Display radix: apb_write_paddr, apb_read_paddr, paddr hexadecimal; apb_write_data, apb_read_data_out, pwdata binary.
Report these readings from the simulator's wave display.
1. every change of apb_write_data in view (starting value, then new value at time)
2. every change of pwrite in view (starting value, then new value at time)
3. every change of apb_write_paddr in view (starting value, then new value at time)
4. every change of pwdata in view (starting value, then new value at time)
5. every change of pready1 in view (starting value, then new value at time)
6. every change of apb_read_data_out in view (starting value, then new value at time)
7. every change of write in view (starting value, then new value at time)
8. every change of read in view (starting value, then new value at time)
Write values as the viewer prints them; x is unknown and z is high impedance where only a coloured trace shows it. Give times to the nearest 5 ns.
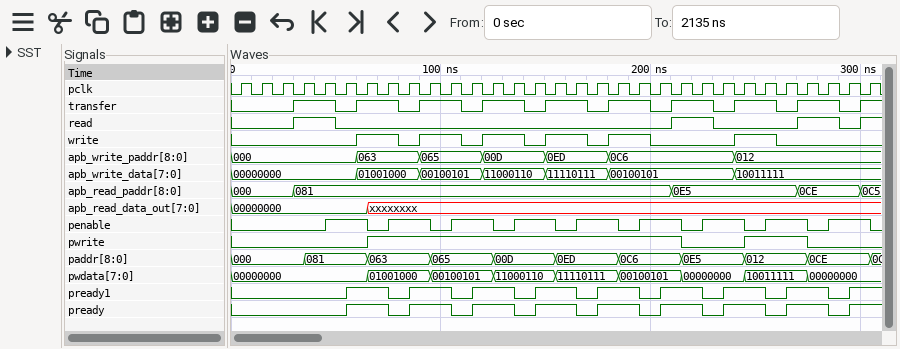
00000000, 01001000 at 60 ns, 00100101 at 90 ns, 11000110 at 120 ns, 11110111 at 150 ns, 00100101 at 180 ns, 10011111 at 240 ns
0, 1 at 65 ns, 0 at 215 ns, 1 at 245 ns, 0 at 275 ns
000, 063 at 60 ns, 065 at 90 ns, 00D at 120 ns, 0ED at 150 ns, 0C6 at 180 ns, 012 at 240 ns
00000000, 01001000 at 65 ns, 00100101 at 95 ns, 11000110 at 125 ns, 11110111 at 155 ns, 00100101 at 185 ns, 00000000 at 215 ns, 10011111 at 245 ns, 00000000 at 275 ns
0, 1 at 55 ns, 0 at 75 ns, 1 at 85 ns, 0 at 105 ns, 1 at 115 ns, 0 at 135 ns, 1 at 145 ns, 0 at 165 ns, 1 at 175 ns, 0 at 195 ns, 1 at 205 ns, 0 at 225 ns, 1 at 235 ns, 0 at 255 ns, 1 at 265 ns, 0 at 285 ns, 1 at 295 ns
00000000, xxxxxxxx at 65 ns
0, 1 at 60 ns, 0 at 80 ns, 1 at 90 ns, 0 at 110 ns, 1 at 120 ns, 0 at 140 ns, 1 at 150 ns, 0 at 170 ns, 1 at 180 ns, 0 at 200 ns, 1 at 240 ns, 0 at 260 ns
0, 1 at 30 ns, 0 at 50 ns, 1 at 210 ns, 0 at 230 ns, 1 at 270 ns, 0 at 290 ns, 1 at 300 ns
